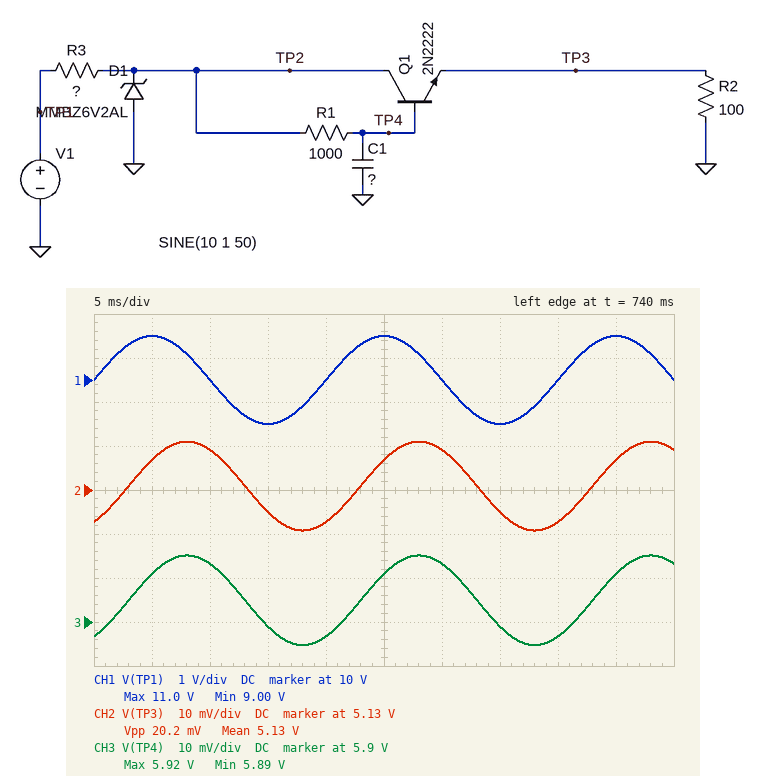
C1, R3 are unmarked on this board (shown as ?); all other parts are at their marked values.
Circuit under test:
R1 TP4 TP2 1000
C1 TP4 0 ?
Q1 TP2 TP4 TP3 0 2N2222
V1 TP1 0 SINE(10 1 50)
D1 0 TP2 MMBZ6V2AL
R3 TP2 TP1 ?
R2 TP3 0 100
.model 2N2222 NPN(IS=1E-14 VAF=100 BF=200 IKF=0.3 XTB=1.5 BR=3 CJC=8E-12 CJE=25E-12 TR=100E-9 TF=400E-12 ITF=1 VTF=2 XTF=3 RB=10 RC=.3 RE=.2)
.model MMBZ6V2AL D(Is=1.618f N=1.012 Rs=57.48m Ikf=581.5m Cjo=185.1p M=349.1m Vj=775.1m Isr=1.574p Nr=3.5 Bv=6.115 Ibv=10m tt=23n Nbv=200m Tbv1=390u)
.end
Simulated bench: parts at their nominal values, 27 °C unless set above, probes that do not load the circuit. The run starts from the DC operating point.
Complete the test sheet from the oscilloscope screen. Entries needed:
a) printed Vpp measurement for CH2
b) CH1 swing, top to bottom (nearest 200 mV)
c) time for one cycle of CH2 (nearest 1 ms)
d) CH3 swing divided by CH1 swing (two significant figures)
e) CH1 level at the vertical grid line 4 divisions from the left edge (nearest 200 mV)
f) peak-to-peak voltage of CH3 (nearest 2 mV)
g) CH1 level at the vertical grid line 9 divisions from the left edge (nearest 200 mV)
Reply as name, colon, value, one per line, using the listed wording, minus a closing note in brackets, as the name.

printed Vpp measurement for CH2: 20.2 mV
CH1 swing, top to bottom: 2.0 V
time for one cycle of CH2: 20 ms
CH3 swing divided by CH1 swing: 0.010
CH1 level at the vertical grid line 4 divisions from the left edge: 10.0 V
peak-to-peak voltage of CH3: 20 mV
CH1 level at the vertical grid line 9 divisions from the left edge: 11.0 V
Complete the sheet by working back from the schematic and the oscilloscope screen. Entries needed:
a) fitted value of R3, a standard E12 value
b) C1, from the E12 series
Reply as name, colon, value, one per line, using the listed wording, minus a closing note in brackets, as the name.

fitted value of R3, a standard E12 value: 3.3 Ω
C1, from the E12 series: 4.7 µF
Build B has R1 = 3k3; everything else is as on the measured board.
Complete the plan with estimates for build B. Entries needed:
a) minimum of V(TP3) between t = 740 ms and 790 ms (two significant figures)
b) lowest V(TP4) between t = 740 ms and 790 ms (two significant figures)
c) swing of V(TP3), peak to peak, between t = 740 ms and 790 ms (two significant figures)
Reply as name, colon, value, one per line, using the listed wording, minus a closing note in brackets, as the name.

minimum of V(TP3) between t = 740 ms and 790 ms: 4.6 V
lowest V(TP4) between t = 740 ms and 790 ms: 5.3 V
swing of V(TP3), peak to peak, between t = 740 ms and 790 ms: 7.4 mV
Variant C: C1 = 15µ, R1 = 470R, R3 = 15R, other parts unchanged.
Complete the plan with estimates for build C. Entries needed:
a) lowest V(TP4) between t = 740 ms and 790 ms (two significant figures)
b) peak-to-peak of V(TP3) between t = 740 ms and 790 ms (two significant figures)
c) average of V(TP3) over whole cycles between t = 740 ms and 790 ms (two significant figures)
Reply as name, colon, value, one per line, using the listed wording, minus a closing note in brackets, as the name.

lowest V(TP4) between t = 740 ms and 790 ms: 6.0 V
peak-to-peak of V(TP3) between t = 740 ms and 790 ms: 4.5 mV
average of V(TP3) over whole cycles between t = 740 ms and 790 ms: 5.2 V
